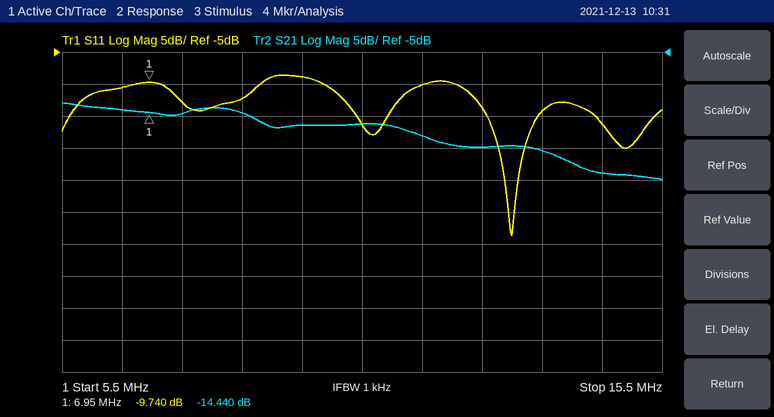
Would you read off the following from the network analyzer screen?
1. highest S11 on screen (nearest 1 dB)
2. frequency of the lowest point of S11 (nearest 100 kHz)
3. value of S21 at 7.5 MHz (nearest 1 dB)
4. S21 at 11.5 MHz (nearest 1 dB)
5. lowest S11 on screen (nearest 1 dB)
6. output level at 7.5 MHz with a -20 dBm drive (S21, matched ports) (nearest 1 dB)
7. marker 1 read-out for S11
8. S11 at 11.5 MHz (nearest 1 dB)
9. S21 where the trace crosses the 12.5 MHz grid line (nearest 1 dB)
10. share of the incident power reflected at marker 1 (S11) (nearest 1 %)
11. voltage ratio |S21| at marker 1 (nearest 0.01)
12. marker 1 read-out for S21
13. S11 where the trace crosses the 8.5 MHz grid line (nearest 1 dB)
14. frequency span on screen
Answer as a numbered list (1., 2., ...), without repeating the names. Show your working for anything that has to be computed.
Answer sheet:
1. -9 dB
2. 13.0 MHz
3. -15 dB
4. -18 dB
5. -34 dB
6. -20 dBm + (-15 dB) = -35 dBm
7. -9.740 dB
8. -10 dB
9. -20 dB
10. 10^(-9.74/10) ≈ 11 %
11. 10^(-14.44/20) ≈ 0.19
12. -14.440 dB
13. -12 dB
14. 10 MHz
